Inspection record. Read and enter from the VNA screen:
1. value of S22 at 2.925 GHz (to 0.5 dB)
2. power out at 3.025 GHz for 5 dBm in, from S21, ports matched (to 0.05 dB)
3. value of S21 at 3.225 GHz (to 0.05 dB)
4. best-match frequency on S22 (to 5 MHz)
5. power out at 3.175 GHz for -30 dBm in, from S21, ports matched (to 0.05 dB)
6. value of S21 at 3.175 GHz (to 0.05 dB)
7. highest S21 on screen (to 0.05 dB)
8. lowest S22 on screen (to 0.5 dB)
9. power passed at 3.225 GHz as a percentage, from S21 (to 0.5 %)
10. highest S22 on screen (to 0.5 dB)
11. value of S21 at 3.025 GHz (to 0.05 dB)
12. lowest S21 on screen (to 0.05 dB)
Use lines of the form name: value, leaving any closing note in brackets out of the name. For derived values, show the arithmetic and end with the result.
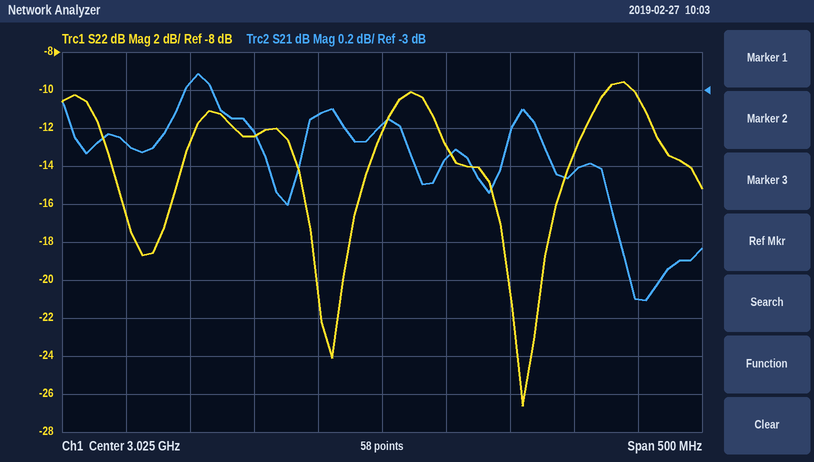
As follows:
value of S22 at 2.925 GHz: -12.5 dB
power out at 3.025 GHz for 5 dBm in, from S21, ports matched: 5 dBm + (-3.20 dB) = 1.80 dBm
value of S21 at 3.225 GHz: -4.10 dB
best-match frequency on S22: 3.135 GHz
power out at 3.175 GHz for -30 dBm in, from S21, ports matched: -30 dBm + (-3.45 dB) = -33.45 dBm
value of S21 at 3.175 GHz: -3.45 dB
highest S21 on screen: -2.90 dB
lowest S22 on screen: -26.5 dB
power passed at 3.225 GHz as a percentage, from S21: 10^(-4.1/10) ≈ 38.9 %, so 39.0 % to the nearest 0.5 %
highest S22 on screen: -9.5 dB
value of S21 at 3.025 GHz: -3.20 dB
lowest S21 on screen: -4.10 dB
